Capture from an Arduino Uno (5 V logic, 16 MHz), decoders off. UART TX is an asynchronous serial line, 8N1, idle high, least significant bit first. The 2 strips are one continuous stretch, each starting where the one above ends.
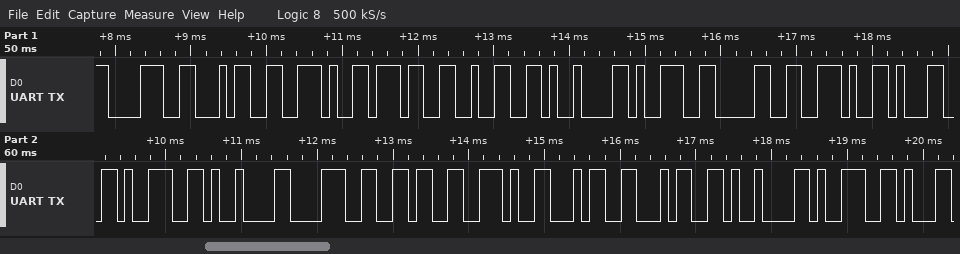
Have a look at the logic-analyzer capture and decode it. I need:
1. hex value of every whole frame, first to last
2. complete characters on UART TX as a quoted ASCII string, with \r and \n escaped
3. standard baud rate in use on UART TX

38 34 2E 37 32 09 39 30 2E 31 39 09 38 36 2E 34 34 09 39
"84.72\t90.19\t86.44\t9"
9600 baud
